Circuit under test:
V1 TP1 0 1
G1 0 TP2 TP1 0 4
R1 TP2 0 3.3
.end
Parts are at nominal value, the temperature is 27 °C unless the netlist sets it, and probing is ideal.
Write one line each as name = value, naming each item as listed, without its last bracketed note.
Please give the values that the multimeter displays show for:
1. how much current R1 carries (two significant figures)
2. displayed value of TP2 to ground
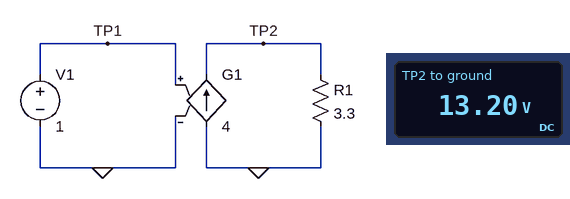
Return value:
how much current R1 carries = 4.0 A
displayed value of TP2 to ground = 13.20 V
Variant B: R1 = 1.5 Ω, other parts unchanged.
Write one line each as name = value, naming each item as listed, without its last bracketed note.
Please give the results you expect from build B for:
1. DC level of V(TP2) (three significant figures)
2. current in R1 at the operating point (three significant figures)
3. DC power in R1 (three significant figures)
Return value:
DC level of V(TP2) = 6.00 V
current in R1 at the operating point = 4.00 A
DC power in R1 = 24.0 W
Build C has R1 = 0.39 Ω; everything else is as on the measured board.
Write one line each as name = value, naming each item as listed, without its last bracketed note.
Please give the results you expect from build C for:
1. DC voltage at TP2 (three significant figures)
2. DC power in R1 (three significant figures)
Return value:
DC voltage at TP2 = 1.56 V
DC power in R1 = 6.24 W
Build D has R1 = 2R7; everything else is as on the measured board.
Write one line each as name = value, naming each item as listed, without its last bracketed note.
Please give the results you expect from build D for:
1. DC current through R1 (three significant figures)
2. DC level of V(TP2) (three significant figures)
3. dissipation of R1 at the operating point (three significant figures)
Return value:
DC current through R1 = 4.00 A
DC level of V(TP2) = 10.8 V
dissipation of R1 at the operating point = 43.2 W
